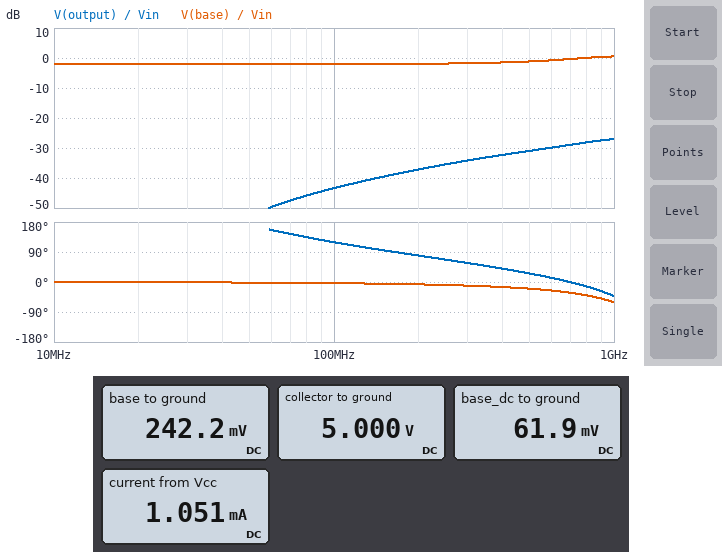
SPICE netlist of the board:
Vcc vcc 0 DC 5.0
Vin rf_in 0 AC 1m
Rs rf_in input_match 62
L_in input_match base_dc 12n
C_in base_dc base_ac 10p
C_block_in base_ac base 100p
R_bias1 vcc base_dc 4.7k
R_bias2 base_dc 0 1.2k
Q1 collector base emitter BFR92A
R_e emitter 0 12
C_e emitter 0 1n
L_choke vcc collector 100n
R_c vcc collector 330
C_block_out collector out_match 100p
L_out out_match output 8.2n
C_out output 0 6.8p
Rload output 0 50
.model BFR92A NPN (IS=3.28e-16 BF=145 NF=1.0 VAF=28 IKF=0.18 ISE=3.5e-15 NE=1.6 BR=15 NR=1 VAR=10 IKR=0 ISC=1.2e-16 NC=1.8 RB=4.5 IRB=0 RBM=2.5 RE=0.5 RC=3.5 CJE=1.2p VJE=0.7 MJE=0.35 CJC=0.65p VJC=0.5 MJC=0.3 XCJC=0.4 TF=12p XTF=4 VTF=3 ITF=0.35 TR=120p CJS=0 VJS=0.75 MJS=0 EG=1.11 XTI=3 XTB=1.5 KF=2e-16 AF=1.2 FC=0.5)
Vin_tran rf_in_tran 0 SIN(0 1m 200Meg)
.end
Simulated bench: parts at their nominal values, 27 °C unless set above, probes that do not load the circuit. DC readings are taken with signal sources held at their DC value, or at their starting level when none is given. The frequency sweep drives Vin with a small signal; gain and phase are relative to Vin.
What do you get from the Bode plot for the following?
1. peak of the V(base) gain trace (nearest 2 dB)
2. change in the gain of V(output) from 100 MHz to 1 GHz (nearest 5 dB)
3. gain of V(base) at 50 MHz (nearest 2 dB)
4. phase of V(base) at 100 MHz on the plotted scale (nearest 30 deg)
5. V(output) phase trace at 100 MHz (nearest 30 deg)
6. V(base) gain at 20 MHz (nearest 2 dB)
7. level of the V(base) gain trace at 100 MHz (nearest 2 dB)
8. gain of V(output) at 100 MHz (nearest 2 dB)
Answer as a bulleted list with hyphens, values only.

- 0 dB
- 15 dB
- -2 dB
- 0 deg
- 120 deg
- -2 dB
- -2 dB
- -44 dB
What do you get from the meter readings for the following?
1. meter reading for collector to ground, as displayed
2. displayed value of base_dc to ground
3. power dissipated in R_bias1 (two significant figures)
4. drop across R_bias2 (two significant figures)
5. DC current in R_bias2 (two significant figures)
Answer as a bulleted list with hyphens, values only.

- 5.000 V
- 61.9 mV
- 5.2 mW
- 62 mV
- 52 µA
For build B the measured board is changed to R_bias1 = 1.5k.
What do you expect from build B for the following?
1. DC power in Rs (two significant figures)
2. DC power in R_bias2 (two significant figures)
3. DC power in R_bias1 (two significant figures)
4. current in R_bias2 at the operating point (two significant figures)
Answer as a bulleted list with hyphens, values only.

- 580 µW
- 30 µW
- 15 mW
- 160 µA
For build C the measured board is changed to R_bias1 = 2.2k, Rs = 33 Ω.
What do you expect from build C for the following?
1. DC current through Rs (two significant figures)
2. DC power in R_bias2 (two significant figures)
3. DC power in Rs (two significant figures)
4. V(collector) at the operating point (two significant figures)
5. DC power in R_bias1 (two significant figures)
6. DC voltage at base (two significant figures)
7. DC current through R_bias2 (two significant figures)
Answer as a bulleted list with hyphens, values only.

- 2.2 mA
- 4.3 µW
- 160 µW
- 5.0 V
- 11 mW
- 250 mV
- 60 µA
